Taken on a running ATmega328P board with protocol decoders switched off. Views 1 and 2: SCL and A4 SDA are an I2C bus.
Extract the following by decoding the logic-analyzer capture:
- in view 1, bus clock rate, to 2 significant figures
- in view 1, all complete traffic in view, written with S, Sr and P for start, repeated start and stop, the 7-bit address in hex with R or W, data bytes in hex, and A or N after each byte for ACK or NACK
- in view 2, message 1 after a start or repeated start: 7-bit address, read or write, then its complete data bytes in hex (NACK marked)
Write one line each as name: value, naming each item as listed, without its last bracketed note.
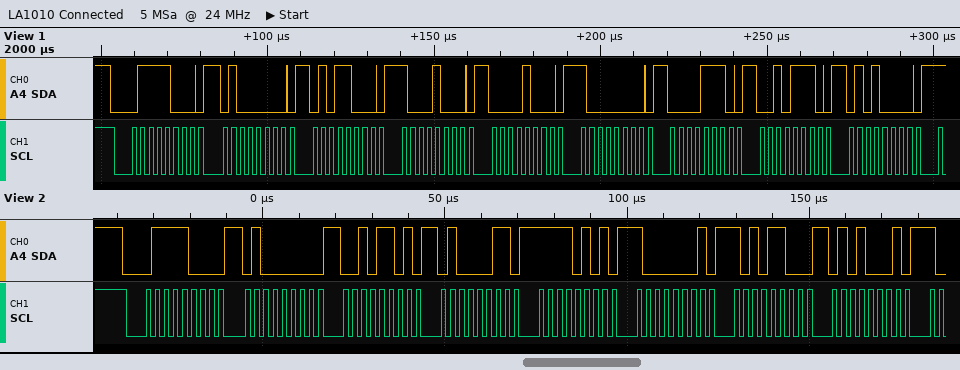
in view 1, bus clock rate, to 2 significant figures: 400 kHz
in view 1, all complete traffic in view, written with S, Sr and P for start, repeated start and stop, the 7-bit address in hex with R or W, data bytes in hex, and A or N after each byte for ACK or NACK: S 3CW A 40 A 58 A 88 A 08 A 80 A 0E A 2E A 50 A
in view 2, message 1 after a start or repeated start: 7-bit address, read or write, then its complete data bytes in hex: 0x3C write: 40 2D 43 F5 81 AC 51
